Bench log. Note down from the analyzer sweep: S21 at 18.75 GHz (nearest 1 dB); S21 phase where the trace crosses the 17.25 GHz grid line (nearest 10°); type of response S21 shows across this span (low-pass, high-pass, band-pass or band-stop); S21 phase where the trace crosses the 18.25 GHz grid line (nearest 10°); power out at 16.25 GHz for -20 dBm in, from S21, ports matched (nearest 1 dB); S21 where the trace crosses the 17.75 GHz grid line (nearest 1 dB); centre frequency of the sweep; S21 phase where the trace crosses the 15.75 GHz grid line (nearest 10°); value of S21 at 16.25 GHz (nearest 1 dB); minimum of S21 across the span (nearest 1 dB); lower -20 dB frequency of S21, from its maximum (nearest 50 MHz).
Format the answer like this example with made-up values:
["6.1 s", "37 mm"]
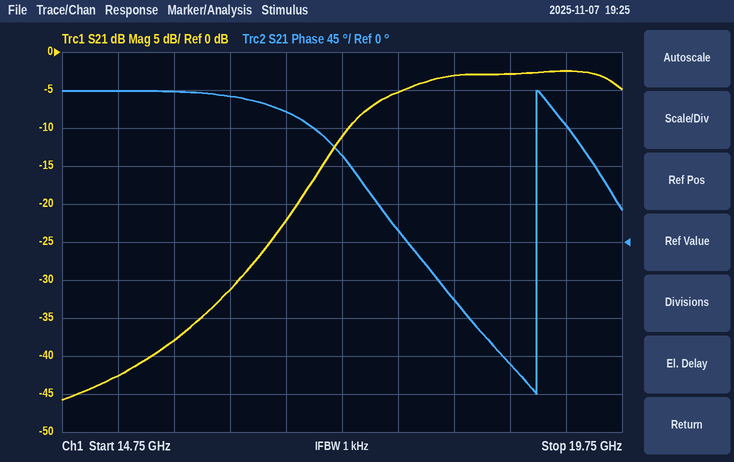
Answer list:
["-3 dB", "100°", "high-pass", "-70°", "-51 dBm", "-5 dB", "17.25 GHz", "180°", "-31 dB", "-46 dB", "16.75 GHz"]
